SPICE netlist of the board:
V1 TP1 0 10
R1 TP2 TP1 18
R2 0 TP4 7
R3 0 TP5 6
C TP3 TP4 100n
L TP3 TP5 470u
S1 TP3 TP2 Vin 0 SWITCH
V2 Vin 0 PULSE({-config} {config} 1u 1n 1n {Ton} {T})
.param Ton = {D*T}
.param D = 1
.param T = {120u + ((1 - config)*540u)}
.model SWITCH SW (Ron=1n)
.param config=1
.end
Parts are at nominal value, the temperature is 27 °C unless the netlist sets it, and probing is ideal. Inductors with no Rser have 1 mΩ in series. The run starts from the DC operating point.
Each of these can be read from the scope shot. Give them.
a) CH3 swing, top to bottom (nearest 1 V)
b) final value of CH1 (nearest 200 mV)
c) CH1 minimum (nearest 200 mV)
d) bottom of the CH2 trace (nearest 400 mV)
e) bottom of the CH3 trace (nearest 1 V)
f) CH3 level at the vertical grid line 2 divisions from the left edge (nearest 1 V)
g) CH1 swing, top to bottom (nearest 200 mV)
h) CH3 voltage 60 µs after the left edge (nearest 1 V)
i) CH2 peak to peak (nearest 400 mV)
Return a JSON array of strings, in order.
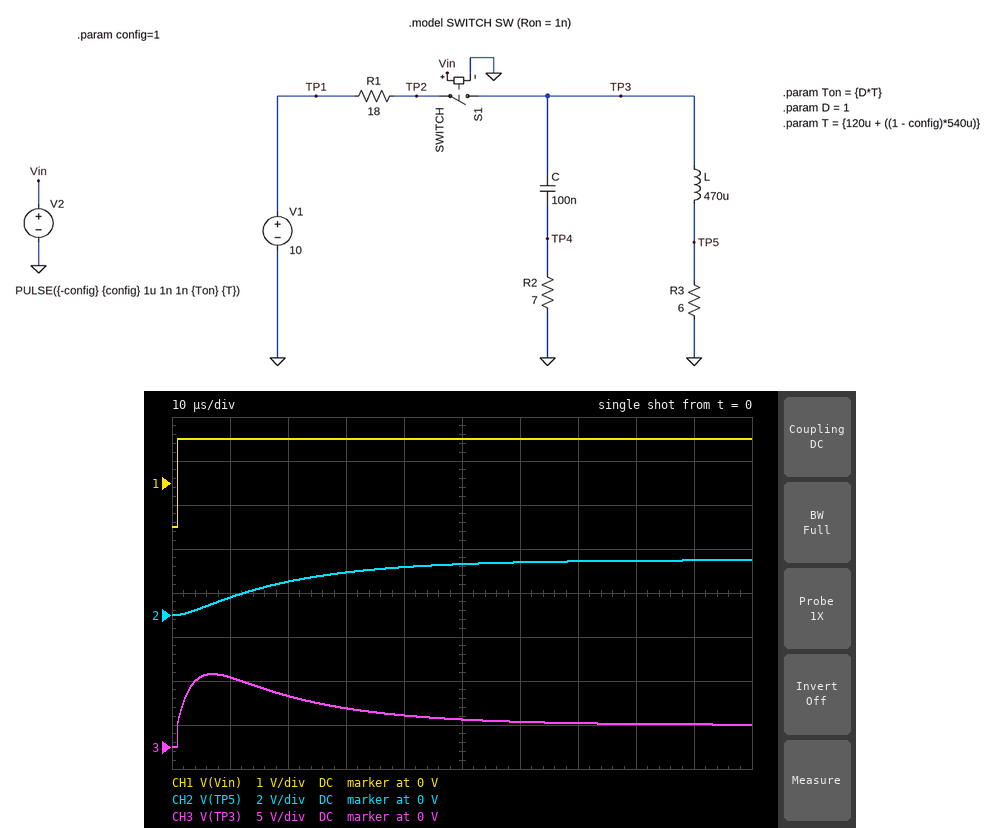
["8 V", "1.0 V", "-1.0 V", "0 V", "0 V", "6 V", "2.0 V", "3 V", "2.4 V"]
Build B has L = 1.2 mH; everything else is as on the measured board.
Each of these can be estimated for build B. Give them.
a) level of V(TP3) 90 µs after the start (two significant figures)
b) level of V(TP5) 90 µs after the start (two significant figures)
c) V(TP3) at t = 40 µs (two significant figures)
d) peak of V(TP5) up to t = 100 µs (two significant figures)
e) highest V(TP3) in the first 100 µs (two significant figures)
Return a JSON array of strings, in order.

["3.8 V", "2.1 V", "6.1 V", "2.2 V", "9.0 V"]
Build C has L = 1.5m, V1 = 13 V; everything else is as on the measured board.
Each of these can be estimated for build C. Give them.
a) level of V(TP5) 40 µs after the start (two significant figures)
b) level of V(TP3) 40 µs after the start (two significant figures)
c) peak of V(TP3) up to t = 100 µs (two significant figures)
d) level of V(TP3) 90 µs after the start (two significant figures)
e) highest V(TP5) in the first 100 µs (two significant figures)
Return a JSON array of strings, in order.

["1.5 V", "8.7 V", "12 V", "5.7 V", "2.6 V"]
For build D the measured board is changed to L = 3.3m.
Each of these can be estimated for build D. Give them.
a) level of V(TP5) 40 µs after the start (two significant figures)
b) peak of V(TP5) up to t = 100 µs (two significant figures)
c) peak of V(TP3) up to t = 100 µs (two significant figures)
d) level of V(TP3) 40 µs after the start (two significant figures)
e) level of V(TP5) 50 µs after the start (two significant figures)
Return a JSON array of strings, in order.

["600 mV", "1.3 V", "9.5 V", "8.3 V", "730 mV"]
